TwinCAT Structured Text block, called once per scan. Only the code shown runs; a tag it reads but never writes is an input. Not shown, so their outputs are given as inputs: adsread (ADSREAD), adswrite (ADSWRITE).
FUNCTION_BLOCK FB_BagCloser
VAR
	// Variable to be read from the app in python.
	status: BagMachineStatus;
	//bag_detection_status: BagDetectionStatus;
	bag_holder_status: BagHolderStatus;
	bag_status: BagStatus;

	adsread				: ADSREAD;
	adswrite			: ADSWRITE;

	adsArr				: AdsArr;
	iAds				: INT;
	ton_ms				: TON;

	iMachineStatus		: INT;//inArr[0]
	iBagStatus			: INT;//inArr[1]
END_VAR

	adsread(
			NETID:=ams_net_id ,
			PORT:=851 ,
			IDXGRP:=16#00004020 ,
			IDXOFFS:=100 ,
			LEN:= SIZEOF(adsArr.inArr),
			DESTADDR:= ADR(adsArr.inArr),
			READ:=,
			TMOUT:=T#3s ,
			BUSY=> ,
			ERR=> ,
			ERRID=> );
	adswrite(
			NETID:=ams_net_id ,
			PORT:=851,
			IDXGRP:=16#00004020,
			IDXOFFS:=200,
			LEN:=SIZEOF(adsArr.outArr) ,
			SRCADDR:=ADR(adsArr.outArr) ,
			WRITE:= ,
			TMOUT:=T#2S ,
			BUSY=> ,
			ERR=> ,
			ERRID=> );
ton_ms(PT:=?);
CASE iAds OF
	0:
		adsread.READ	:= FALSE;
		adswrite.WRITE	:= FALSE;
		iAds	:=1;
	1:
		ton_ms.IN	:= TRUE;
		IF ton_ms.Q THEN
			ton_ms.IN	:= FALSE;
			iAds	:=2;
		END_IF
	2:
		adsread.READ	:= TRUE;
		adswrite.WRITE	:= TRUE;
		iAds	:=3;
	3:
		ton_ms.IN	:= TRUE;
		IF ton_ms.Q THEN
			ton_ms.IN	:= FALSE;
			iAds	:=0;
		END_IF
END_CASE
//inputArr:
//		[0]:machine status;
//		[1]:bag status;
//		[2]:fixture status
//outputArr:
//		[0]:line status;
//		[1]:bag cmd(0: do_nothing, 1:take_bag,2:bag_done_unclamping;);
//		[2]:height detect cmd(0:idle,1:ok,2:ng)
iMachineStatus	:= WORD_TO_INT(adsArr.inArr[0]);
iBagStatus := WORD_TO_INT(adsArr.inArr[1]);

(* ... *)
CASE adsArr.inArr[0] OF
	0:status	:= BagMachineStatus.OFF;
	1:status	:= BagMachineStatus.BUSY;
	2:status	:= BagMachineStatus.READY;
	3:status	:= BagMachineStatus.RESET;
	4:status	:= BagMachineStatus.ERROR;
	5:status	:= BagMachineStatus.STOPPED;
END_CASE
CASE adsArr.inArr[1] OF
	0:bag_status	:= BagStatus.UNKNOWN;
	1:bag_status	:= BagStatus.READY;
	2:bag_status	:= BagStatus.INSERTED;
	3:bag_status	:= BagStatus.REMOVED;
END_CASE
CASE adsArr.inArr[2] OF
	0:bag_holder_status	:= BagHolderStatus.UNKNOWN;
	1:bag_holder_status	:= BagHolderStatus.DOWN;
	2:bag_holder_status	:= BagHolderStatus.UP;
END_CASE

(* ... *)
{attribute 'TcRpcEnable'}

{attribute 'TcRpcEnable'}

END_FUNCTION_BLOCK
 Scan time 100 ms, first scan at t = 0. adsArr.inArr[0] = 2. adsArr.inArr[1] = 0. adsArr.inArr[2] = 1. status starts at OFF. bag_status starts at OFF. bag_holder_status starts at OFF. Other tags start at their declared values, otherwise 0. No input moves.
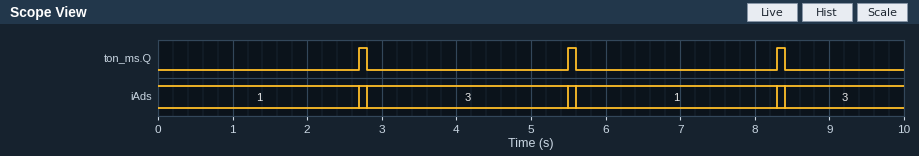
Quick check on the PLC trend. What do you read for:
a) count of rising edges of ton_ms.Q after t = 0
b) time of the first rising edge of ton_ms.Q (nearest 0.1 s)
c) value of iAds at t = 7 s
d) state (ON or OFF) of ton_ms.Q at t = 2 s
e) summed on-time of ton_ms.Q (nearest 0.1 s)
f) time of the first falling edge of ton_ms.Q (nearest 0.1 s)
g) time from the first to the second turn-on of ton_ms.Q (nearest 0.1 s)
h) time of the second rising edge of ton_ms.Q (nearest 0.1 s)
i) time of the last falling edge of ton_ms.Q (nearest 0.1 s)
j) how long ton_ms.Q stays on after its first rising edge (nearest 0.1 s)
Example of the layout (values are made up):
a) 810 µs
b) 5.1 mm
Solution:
a) 3
b) 2.7 s
c) 1
d) OFF
e) 0.3 s
f) 2.8 s
g) 2.8 s
h) 5.5 s
i) 8.4 s
j) 0.1 s
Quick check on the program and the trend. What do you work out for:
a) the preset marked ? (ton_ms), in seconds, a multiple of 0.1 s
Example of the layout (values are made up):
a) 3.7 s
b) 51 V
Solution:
a) 2.5 s
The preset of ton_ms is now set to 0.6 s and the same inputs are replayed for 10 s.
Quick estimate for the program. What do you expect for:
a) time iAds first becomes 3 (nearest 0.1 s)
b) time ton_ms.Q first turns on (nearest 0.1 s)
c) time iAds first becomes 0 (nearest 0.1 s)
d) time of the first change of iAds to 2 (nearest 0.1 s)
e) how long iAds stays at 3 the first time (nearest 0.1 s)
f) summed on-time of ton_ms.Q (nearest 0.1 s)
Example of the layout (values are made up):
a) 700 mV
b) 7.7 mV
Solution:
a) 0.9 s
b) 0.8 s
c) 1.7 s
d) 0.8 s
e) 0.8 s
f) 1.1 s
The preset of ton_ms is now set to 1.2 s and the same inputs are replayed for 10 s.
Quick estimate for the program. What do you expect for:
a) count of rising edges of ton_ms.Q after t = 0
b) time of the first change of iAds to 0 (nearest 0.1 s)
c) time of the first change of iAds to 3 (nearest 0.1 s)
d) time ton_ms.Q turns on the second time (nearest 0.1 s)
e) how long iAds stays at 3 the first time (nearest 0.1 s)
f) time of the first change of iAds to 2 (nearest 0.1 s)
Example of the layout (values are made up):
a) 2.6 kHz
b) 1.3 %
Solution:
a) 6
b) 2.9 s
c) 1.5 s
d) 2.9 s
e) 1.4 s
f) 1.4 s
